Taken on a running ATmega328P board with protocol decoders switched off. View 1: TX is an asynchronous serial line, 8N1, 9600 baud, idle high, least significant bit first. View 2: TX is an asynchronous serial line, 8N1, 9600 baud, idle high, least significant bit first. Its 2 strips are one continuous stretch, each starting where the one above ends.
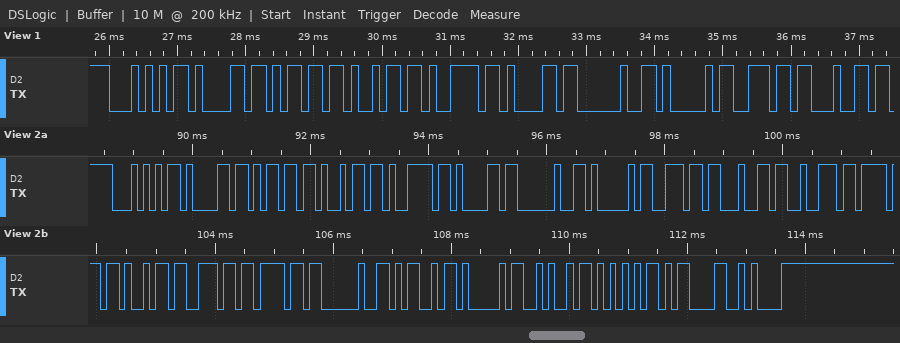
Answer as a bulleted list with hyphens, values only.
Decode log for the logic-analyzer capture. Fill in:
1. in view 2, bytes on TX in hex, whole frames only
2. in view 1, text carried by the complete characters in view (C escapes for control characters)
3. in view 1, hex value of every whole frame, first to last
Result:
- 54 61 6D 69 79 61 20 41 6E 64 72 6F 69 6E 6F 20 4D 41 4A 55 0D 0A
- "Tamiya And"
- 54 61 6D 69 79 61 20 41 6E 64
